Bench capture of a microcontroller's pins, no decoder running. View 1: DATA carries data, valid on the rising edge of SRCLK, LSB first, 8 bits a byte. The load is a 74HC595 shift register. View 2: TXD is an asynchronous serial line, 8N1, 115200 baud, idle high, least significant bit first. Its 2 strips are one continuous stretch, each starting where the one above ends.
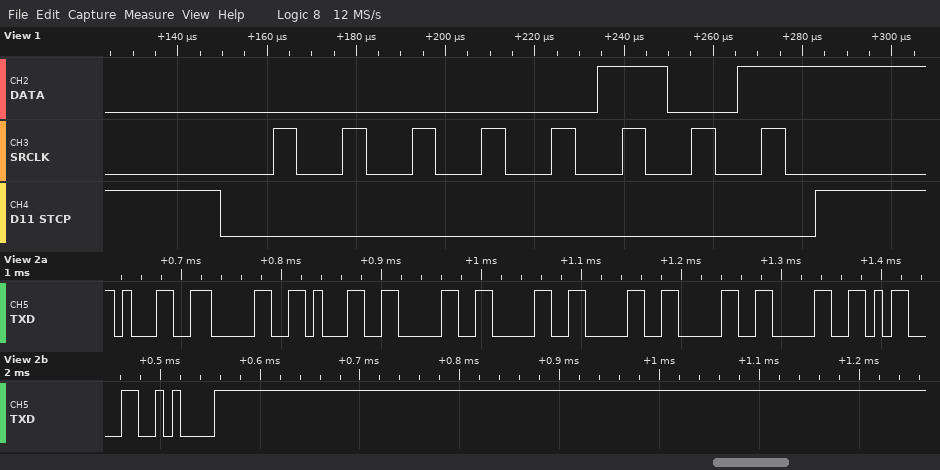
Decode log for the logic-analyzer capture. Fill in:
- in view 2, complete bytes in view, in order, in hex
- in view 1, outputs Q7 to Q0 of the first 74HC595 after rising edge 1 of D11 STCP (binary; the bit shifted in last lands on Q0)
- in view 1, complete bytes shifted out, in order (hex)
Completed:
0x31 0x30 0x31 0x30 0x30 0x30 0x30 0x30 0x0D 0x0A
00000101
A0
